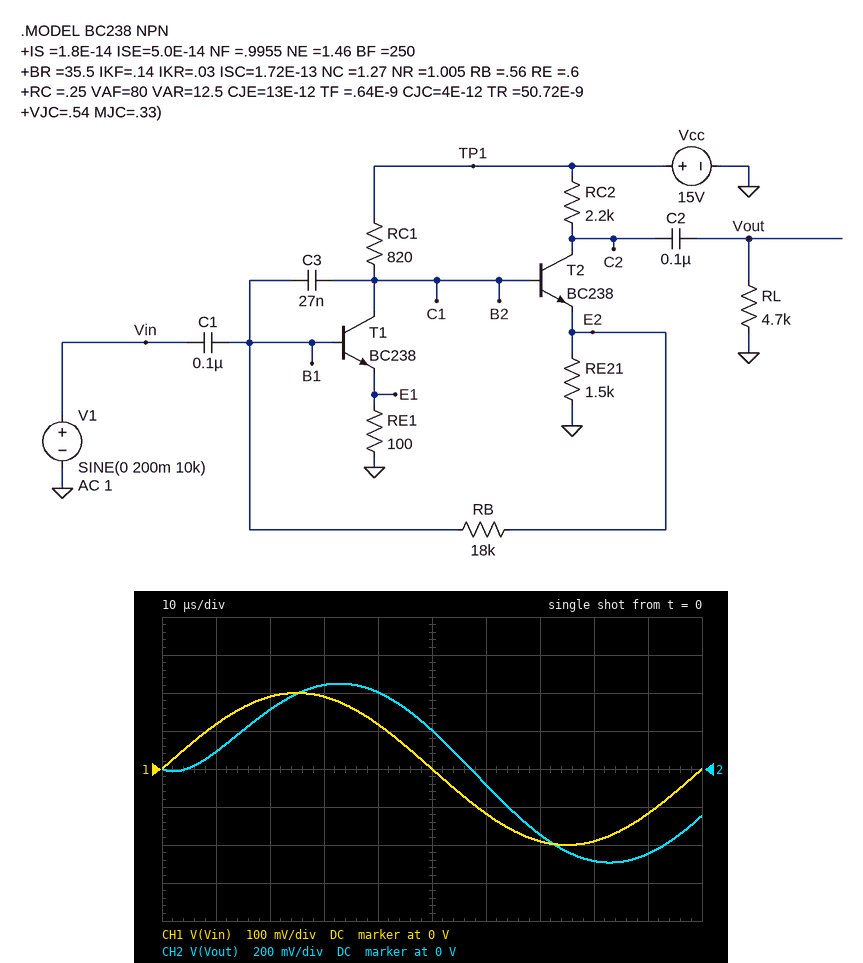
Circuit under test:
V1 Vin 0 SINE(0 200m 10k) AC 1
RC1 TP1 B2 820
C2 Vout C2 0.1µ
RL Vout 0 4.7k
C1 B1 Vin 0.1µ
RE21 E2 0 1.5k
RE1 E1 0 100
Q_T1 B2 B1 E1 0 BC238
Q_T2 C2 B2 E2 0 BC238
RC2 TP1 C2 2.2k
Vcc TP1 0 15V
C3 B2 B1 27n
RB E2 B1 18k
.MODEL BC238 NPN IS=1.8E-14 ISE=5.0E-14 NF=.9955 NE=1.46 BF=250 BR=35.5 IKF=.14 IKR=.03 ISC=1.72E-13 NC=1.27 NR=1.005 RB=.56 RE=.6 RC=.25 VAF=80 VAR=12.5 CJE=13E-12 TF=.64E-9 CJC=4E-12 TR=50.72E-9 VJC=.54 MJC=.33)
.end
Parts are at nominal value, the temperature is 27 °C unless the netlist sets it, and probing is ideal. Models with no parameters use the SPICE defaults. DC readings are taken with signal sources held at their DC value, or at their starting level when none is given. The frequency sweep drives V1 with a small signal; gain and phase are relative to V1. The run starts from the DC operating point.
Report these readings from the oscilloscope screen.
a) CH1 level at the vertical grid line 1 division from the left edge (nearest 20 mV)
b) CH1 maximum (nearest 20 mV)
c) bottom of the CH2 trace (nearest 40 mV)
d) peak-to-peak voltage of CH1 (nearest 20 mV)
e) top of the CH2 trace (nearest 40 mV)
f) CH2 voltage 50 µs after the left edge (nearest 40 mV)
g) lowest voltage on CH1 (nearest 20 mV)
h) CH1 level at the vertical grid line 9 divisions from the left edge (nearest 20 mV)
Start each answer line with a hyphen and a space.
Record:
- 120 mV
- 200 mV
- -480 mV
- 400 mV
- 440 mV
- 200 mV
- -200 mV
- -120 mV
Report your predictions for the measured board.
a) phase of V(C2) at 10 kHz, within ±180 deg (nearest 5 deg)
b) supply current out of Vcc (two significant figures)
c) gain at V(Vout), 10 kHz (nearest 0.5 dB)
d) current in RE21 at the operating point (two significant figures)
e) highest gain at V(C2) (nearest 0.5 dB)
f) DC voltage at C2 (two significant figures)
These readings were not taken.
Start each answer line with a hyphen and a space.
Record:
- -30 deg
- 16 mA
- 7.5 dB
- 2.2 mA
- 8.0 dB
- 10 V
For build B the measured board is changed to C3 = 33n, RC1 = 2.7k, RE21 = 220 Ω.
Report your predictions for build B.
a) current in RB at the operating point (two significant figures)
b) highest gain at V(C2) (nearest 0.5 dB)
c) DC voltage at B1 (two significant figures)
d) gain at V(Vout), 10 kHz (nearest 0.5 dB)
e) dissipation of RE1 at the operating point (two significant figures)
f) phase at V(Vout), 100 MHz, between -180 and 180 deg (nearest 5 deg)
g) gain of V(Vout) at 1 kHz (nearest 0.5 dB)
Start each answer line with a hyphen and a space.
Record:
- 21 µA
- 0 dB
- 1.1 V
- -2.5 dB
- 1.8 mW
- 0 deg
- -3.0 dB
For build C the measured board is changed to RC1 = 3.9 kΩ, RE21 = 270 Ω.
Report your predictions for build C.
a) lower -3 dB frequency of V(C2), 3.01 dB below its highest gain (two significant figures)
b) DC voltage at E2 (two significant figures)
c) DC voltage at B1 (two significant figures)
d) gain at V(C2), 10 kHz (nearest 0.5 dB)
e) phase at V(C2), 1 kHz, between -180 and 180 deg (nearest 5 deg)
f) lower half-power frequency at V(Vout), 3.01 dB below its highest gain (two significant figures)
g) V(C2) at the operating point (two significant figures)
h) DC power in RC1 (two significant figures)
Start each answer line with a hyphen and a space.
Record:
- 190 Hz
- 1.3 V
- 1.0 V
- 24.0 dB
- 5 deg
- 400 Hz
- 4.4 V
- 43 mW
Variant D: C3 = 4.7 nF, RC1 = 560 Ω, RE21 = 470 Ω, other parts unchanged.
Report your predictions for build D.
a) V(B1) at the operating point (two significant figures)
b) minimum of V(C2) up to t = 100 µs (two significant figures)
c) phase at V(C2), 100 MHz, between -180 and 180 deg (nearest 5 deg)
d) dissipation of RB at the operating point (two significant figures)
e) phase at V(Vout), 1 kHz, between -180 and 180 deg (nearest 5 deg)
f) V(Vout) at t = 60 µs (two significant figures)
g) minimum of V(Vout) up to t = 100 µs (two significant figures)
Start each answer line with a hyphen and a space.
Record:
- 2.3 V
- 3.4 V
- 0 deg
- 120 µW
- -145 deg
- 220 mV
- -340 mV
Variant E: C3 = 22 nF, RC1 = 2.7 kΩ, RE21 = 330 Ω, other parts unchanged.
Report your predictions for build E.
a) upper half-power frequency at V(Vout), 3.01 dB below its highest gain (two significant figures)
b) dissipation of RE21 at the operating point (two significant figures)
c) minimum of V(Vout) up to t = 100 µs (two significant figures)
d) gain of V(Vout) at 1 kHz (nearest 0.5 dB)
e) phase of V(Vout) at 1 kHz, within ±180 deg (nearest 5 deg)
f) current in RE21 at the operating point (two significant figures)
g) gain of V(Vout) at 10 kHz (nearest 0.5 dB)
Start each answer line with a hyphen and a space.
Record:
- 20 kHz
- 7.5 mW
- -2.5 V
- 24.0 dB
- 30 deg
- 4.8 mA
- 23.5 dB
